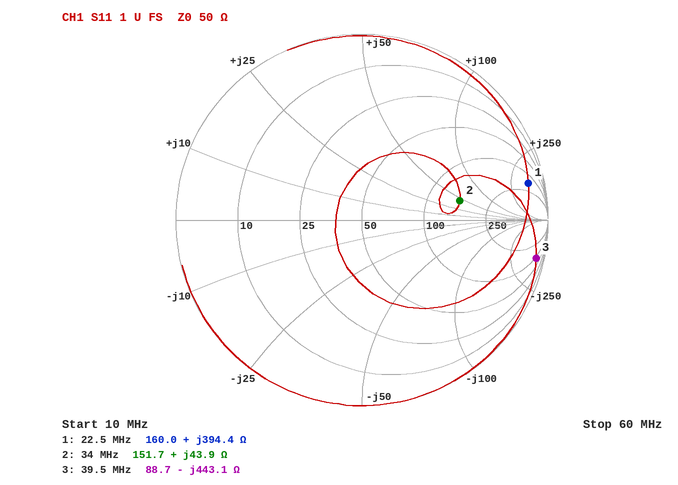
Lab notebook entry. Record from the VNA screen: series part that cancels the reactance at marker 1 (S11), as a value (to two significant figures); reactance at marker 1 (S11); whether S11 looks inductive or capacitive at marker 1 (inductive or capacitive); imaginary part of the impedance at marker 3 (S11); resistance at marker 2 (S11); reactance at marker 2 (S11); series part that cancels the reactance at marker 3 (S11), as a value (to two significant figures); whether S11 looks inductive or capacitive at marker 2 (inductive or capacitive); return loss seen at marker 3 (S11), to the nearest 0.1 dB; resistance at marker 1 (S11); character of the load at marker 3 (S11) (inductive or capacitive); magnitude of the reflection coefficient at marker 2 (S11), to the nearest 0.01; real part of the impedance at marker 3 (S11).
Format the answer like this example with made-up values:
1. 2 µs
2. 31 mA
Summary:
1. 18 pF
2. +394.4 Ω
3. inductive
4. -443.1 Ω
5. 151.7 Ω
6. +43.9 Ω
7. 1.8 µH
8. inductive
9. 0.4 dB
10. 160.0 Ω
11. capacitive
12. 0.54
13. 88.7 Ω
